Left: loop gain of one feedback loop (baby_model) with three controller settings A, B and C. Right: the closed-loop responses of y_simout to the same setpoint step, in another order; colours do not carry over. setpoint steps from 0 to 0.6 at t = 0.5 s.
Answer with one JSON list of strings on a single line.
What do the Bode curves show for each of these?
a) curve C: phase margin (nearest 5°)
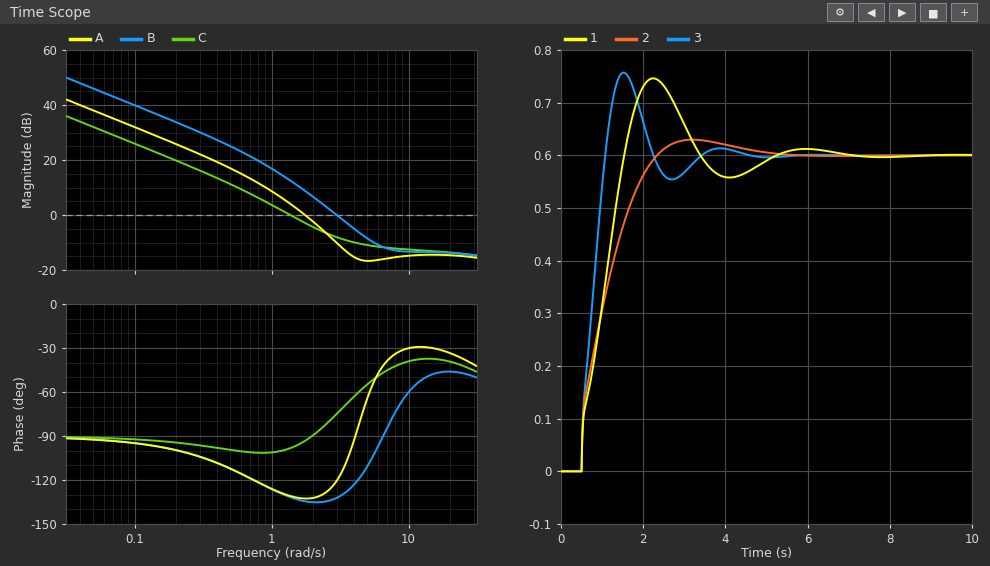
["80°"]
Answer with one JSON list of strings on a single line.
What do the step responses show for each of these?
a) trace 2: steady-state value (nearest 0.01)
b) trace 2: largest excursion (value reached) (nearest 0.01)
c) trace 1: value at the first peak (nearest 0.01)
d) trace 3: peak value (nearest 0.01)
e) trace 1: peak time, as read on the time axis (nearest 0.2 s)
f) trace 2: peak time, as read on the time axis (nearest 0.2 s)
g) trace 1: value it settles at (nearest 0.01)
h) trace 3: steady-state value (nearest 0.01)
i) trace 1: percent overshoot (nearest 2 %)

["0.60", "0.63", "0.75", "0.76", "2.2 s", "3.2 s", "0.60", "0.60", "24 %"]
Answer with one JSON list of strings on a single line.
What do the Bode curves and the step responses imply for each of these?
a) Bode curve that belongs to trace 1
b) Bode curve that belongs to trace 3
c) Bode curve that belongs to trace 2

["A", "B", "C"]
